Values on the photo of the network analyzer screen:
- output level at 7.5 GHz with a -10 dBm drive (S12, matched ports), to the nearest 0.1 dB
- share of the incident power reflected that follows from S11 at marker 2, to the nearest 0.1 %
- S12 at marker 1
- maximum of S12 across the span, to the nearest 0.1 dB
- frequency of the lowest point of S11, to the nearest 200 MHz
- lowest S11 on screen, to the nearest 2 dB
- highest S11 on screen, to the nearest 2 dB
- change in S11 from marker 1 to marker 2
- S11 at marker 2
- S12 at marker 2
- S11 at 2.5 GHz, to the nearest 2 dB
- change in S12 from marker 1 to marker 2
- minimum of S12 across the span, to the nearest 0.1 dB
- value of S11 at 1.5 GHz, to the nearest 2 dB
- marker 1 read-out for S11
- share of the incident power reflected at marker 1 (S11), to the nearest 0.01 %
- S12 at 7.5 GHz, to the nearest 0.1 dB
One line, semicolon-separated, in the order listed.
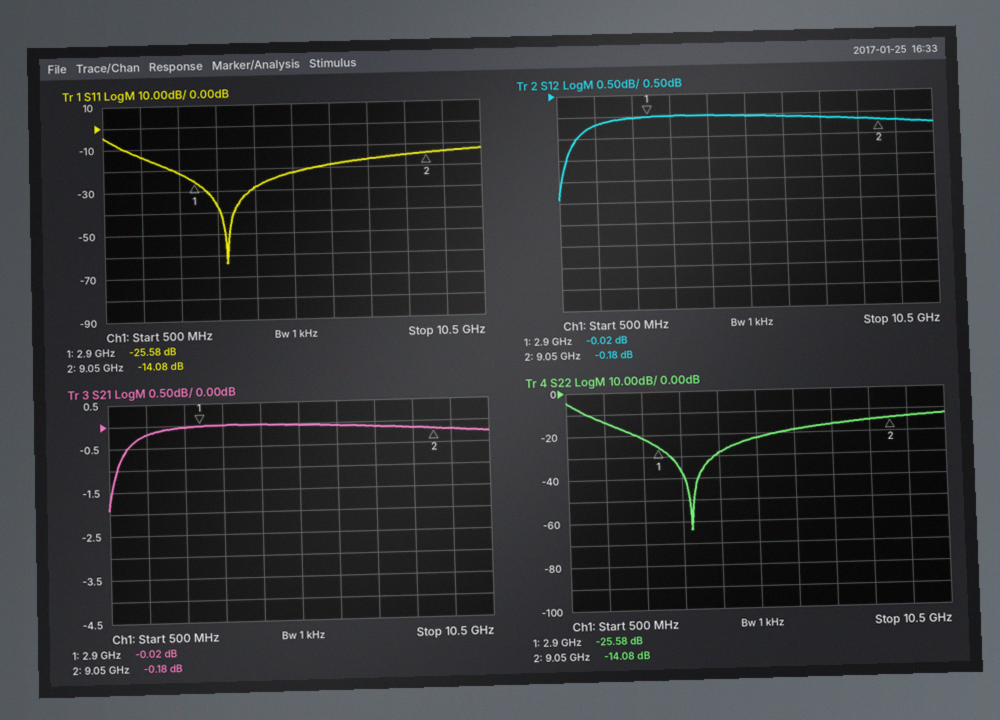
-10.1 dBm; 3.9 %; -0.02 dB; 0.0 dB; 3.8 GHz; -64 dB; -4 dB; 11.50 dB; -14.08 dB; -0.18 dB; -22 dB; -0.16 dB; -1.9 dB; -14 dB; -25.58 dB; 0.28 %; -0.1 dB
